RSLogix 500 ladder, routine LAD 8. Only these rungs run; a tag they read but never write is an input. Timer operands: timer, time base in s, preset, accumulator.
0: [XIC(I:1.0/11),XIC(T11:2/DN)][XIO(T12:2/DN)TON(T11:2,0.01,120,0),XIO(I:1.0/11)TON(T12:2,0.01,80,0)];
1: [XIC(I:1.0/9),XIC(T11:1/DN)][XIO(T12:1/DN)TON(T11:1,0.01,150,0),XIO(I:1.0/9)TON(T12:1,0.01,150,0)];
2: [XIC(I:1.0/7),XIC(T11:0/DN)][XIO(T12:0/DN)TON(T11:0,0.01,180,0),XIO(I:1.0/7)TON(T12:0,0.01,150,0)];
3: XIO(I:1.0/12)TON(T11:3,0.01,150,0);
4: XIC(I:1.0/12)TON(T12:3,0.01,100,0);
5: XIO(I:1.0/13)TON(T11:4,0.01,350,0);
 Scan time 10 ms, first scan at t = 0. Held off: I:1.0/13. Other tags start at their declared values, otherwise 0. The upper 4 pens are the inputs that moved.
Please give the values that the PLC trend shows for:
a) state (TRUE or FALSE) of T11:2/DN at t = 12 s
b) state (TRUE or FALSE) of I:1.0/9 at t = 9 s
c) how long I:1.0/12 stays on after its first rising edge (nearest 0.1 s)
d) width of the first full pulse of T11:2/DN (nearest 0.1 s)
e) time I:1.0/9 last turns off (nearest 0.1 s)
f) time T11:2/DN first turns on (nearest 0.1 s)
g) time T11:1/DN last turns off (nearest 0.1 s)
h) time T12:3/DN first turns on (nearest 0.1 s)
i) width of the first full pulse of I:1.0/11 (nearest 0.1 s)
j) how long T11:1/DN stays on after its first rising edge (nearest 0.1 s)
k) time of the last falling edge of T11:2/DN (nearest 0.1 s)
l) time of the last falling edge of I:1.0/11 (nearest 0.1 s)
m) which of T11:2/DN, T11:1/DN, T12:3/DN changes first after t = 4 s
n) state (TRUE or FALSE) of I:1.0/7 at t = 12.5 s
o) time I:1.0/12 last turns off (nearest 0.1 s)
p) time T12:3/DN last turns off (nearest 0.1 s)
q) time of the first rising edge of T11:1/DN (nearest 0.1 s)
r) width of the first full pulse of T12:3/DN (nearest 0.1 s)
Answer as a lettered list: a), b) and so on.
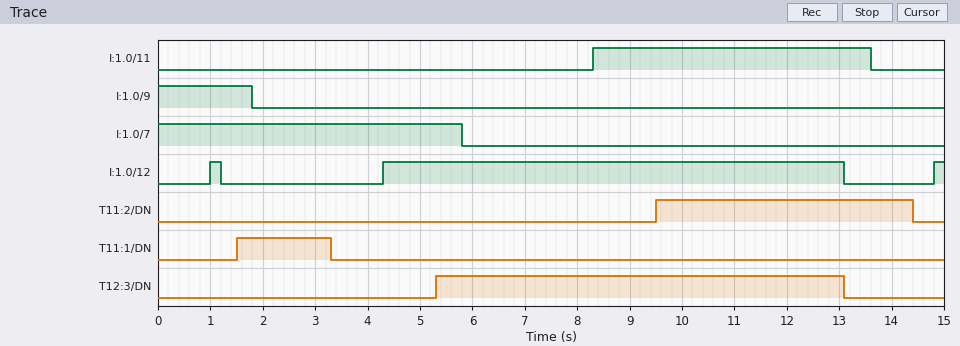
a) TRUE
b) FALSE
c) 0.2 s
d) 4.9 s
e) 1.8 s
f) 9.5 s
g) 3.3 s
h) 5.3 s
i) 5.3 s
j) 1.8 s
k) 14.4 s
l) 13.6 s
m) T12:3/DN
n) FALSE
o) 13.1 s
p) 13.1 s
q) 1.5 s
r) 7.8 s
